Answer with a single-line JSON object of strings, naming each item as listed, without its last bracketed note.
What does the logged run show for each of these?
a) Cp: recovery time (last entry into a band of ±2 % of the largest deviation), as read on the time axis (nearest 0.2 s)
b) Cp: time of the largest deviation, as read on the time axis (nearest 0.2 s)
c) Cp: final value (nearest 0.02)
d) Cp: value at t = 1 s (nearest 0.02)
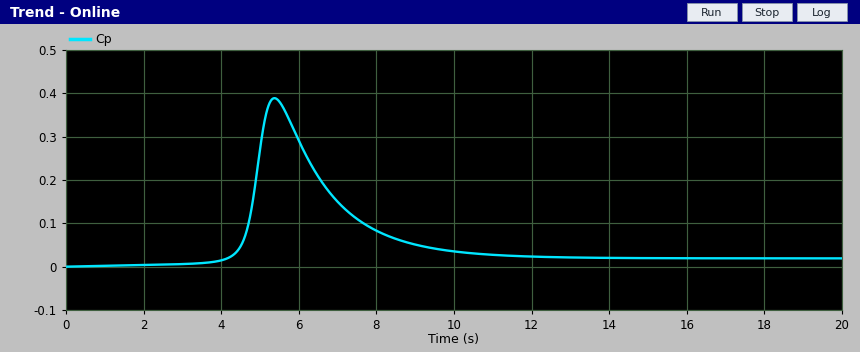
{"Cp: recovery time (last entry into a band of ±2 % of the largest deviation), as read on the time axis": "11.0 s", "Cp: time of the largest deviation, as read on the time axis": "5.4 s", "Cp: final value": "0.02", "Cp: value at t = 1 s": "0.00"}
